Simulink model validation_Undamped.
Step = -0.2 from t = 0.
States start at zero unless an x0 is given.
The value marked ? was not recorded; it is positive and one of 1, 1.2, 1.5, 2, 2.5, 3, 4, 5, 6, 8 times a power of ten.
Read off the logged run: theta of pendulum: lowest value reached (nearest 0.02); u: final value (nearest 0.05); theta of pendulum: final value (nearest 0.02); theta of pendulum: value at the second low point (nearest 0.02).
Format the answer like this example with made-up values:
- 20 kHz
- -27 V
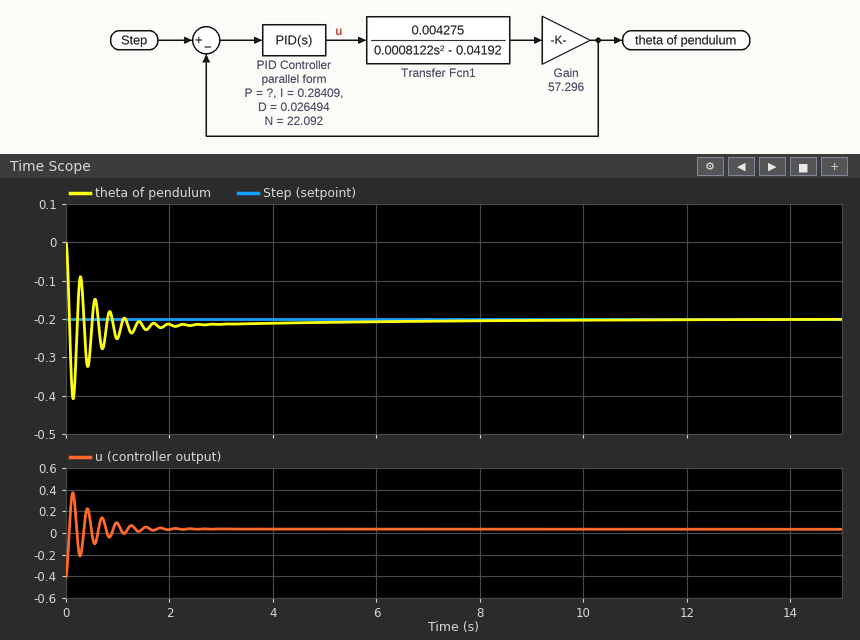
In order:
- -0.40
- 0.05
- -0.20
- -0.32
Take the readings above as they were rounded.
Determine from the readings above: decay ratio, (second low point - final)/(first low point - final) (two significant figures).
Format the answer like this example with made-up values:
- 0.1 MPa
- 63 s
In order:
- 0.60
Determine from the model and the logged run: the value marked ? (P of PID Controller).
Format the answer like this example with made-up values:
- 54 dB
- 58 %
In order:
- 1.5
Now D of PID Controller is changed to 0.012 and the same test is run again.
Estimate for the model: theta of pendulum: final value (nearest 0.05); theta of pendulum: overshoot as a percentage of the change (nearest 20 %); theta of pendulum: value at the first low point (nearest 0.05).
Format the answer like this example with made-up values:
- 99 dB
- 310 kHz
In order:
- -0.20
- 120 %
- -0.45
